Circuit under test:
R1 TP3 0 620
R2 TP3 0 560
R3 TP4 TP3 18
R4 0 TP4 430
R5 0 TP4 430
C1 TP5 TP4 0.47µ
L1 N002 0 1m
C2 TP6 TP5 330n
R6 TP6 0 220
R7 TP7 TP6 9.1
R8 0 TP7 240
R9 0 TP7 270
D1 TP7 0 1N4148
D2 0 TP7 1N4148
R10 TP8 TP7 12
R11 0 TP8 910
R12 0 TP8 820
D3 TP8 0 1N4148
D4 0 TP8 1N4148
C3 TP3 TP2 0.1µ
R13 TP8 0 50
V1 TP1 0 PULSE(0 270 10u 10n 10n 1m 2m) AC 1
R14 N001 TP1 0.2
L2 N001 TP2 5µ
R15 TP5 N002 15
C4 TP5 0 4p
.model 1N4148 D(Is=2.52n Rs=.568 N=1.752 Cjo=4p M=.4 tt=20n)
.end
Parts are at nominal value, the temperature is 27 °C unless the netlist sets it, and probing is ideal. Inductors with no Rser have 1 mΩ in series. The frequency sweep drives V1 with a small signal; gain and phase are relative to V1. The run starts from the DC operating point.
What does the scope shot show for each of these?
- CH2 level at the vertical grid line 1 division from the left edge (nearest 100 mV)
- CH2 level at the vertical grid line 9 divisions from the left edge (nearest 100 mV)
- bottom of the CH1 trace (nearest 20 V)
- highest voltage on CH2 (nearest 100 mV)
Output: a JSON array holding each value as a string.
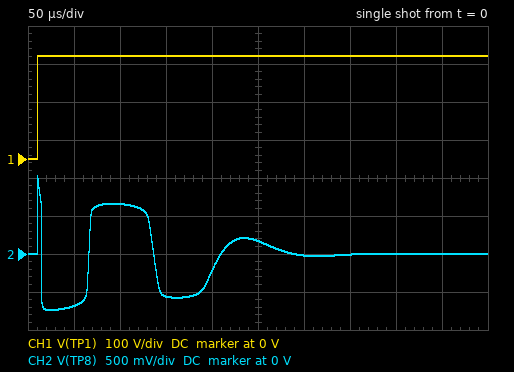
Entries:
["-700 mV", "0 V", "0 V", "1.0 V"]
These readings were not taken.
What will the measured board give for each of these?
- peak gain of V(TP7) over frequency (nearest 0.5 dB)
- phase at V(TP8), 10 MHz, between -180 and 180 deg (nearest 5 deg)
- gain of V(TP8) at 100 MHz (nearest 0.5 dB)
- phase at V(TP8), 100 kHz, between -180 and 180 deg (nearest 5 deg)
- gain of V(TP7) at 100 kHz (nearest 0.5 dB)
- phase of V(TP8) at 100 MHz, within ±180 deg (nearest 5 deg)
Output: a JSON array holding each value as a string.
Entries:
["-5.5 dB", "-85 deg", "-45.0 dB", "25 deg", "-6.0 dB", "-110 deg"]
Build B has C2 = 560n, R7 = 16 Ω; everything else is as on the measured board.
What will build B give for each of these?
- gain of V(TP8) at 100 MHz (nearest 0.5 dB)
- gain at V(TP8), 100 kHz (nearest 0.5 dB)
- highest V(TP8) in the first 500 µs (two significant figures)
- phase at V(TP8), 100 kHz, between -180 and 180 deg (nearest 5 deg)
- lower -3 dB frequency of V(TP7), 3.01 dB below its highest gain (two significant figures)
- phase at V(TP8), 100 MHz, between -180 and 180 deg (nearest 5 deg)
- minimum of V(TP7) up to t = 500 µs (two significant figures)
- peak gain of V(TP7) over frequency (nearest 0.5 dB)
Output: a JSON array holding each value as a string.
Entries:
["-45.5 dB", "-9.0 dB", "980 mV", "20 deg", "37 kHz", "-110 deg", "-1.1 V", "-6.5 dB"]
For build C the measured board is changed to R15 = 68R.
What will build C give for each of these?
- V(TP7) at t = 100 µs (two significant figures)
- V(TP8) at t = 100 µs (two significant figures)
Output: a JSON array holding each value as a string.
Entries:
["570 mV", "450 mV"]
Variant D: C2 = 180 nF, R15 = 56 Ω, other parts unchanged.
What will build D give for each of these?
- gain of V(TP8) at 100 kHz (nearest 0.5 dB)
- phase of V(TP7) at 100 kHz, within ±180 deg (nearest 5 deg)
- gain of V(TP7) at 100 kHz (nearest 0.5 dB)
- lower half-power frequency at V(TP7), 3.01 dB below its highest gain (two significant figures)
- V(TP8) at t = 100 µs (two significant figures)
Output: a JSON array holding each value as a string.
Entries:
["-8.5 dB", "30 deg", "-6.5 dB", "48 kHz", "520 mV"]
